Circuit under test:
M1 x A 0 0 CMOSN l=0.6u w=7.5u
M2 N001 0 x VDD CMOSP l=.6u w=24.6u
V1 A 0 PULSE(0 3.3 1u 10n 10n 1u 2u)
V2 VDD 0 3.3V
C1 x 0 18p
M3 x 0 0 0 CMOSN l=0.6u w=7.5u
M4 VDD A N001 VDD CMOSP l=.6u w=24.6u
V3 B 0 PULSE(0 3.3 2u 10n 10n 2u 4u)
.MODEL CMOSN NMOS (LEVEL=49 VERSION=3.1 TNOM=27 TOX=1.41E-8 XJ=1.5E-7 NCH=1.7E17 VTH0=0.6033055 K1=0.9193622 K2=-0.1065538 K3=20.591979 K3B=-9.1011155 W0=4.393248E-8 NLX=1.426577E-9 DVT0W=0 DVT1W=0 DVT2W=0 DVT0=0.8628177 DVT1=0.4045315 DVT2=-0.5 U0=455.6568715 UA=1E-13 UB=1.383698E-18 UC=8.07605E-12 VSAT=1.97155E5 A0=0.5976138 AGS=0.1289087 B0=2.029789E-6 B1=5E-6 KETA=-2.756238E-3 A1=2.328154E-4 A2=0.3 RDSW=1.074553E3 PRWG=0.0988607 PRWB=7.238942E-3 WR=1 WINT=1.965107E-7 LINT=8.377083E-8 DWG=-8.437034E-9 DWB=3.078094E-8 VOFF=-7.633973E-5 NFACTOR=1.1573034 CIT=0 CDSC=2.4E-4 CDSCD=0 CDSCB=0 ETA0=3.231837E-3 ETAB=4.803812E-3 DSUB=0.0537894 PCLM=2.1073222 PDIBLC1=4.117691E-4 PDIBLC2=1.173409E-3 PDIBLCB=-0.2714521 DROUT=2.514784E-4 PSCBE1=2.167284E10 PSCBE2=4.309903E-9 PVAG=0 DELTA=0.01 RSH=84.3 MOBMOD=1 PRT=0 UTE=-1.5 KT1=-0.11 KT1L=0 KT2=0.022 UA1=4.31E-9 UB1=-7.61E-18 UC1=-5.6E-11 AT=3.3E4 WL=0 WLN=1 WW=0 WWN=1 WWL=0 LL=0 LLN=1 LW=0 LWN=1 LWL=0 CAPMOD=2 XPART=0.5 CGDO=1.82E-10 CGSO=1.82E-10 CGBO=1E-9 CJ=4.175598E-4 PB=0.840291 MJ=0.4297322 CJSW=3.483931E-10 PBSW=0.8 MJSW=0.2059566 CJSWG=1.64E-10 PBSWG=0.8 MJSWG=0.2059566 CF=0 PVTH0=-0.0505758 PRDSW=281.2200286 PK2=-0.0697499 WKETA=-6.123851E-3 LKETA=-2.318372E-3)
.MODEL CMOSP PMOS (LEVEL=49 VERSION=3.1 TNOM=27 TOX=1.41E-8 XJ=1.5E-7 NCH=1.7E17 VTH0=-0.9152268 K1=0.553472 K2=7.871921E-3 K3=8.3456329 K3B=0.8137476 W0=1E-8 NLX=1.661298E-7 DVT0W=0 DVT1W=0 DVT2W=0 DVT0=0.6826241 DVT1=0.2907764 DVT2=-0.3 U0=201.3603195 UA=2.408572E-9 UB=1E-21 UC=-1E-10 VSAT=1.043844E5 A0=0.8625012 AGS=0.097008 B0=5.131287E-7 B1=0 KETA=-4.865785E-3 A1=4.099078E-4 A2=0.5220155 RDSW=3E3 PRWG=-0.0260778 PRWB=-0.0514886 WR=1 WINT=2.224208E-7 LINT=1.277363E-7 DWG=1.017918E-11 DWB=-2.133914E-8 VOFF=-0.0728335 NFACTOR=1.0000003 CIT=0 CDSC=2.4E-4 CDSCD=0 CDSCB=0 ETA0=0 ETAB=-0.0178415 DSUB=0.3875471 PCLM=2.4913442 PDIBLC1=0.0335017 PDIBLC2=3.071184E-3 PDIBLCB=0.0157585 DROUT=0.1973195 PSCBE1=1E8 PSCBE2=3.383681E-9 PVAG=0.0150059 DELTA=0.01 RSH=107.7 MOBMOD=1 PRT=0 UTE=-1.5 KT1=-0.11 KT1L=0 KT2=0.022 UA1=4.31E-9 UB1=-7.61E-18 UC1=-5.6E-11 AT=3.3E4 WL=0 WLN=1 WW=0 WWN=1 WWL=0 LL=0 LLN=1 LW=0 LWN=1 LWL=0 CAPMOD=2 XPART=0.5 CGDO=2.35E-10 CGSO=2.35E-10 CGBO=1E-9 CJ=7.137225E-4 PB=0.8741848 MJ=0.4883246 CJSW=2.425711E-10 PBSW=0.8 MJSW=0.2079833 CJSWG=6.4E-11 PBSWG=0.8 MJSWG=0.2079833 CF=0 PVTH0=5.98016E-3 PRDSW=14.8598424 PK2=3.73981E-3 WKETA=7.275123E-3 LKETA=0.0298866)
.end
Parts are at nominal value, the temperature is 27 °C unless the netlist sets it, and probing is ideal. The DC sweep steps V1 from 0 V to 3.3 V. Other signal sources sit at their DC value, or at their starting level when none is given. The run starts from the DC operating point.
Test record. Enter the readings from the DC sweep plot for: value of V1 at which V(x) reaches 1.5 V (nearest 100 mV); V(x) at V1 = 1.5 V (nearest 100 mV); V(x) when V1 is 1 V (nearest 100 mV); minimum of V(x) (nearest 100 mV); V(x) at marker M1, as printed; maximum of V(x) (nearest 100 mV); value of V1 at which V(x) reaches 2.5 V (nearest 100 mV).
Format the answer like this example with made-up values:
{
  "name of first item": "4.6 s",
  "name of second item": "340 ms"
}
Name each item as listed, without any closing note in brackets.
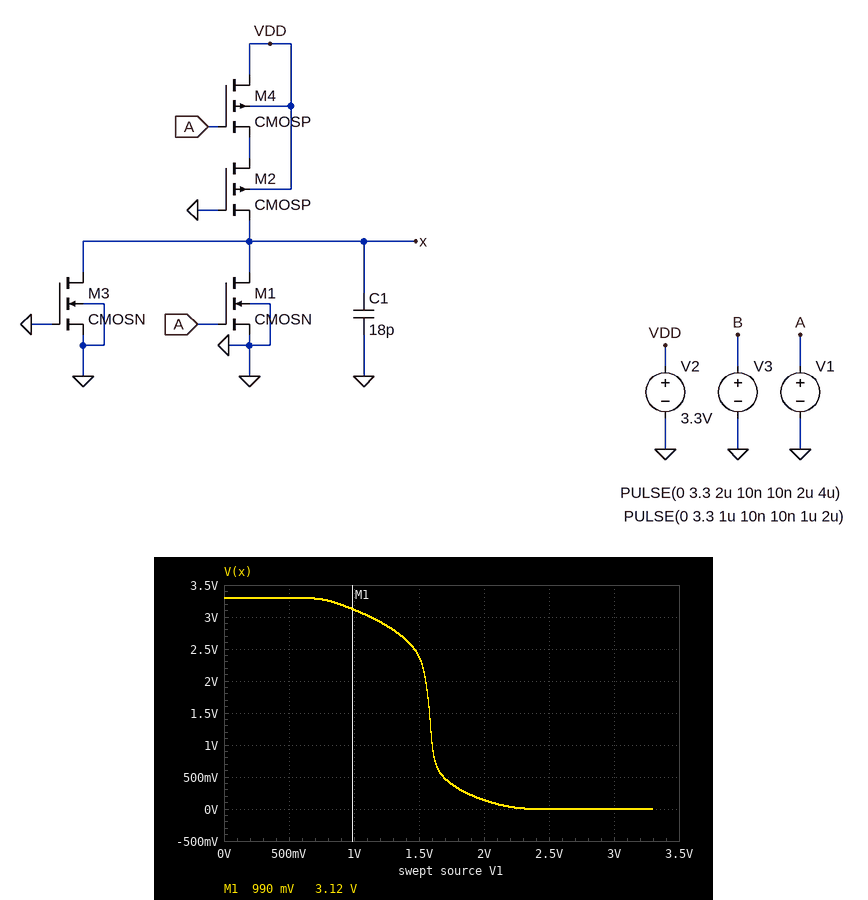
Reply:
{
  "value of V1 at which V(x) reaches 1.5 V": "1.6 V",
  "V(x) at V1 = 1.5 V": "2.4 V",
  "V(x) when V1 is 1 V": "3.1 V",
  "minimum of V(x)": "0 V",
  "V(x) at marker M1, as printed": "3.12 V",
  "maximum of V(x)": "3.3 V",
  "value of V1 at which V(x) reaches 2.5 V": "1.5 V"
}
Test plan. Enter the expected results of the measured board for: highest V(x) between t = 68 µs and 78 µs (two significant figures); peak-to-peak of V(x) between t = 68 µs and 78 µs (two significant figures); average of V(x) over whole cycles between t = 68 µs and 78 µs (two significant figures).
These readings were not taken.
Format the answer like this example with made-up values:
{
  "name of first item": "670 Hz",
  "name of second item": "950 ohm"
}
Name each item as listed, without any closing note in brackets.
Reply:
{
  "highest V(x) between t = 68 µs and 78 µs": "3.3 V",
  "peak-to-peak of V(x) between t = 68 µs and 78 µs": "3.3 V",
  "average of V(x) over whole cycles between t = 68 µs and 78 µs": "1.6 V"
}
